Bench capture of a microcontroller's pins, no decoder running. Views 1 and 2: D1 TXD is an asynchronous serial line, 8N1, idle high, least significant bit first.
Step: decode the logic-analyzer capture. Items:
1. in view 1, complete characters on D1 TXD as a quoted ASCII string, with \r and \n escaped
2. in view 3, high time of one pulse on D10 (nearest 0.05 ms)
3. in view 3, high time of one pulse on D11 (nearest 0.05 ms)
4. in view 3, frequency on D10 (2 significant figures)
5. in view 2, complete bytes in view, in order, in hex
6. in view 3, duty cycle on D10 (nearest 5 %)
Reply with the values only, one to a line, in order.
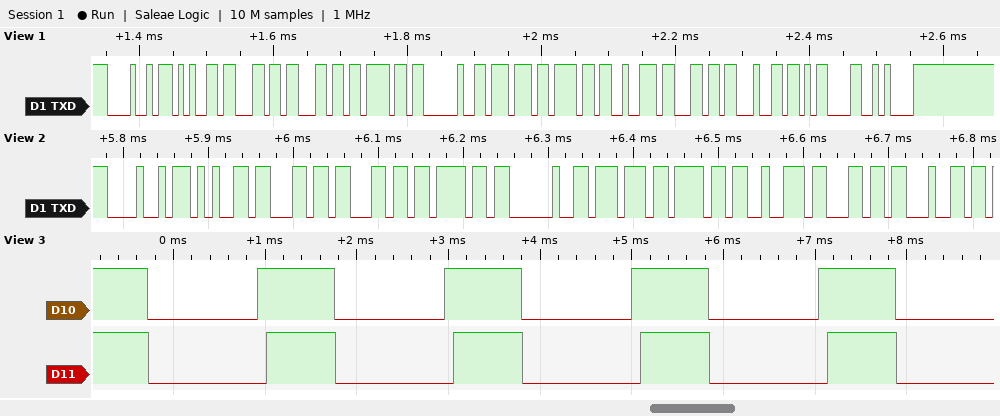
"Hello world\r\n"
0.85 ms
0.75 ms
490 Hz
48 65 6C 6C 6F 20 77 6F 72 6C 64
40 %
